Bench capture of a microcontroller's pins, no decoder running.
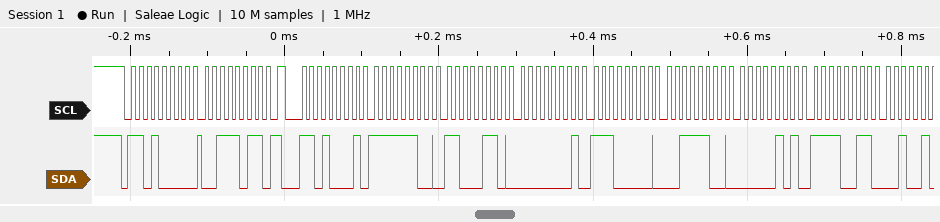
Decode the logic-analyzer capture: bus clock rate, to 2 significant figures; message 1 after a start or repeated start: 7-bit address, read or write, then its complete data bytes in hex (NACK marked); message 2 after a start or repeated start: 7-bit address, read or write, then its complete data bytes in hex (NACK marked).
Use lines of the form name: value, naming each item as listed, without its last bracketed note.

bus clock rate, to 2 significant figures: 100 kHz
message 1 after a start or repeated start: 7-bit address, read or write, then its complete data bytes in hex: 0x68 write: 3B
message 2 after a start or repeated start: 7-bit address, read or write, then its complete data bytes in hex: 0x68 read: FC C6 01 E0 3C 05 F3
